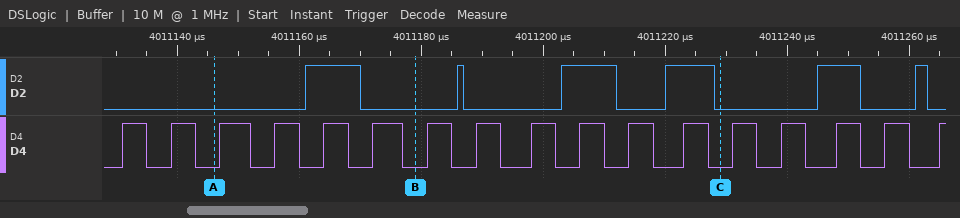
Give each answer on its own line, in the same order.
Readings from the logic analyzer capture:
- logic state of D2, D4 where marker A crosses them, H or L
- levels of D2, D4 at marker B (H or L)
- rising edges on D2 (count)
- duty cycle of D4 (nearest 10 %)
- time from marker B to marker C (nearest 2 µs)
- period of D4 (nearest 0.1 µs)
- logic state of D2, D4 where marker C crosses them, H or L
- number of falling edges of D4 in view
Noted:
D2=L, D4=L
D2=L, D4=L
6
50 %
50 µs
8.4 µs
D2=L, D4=L
16
